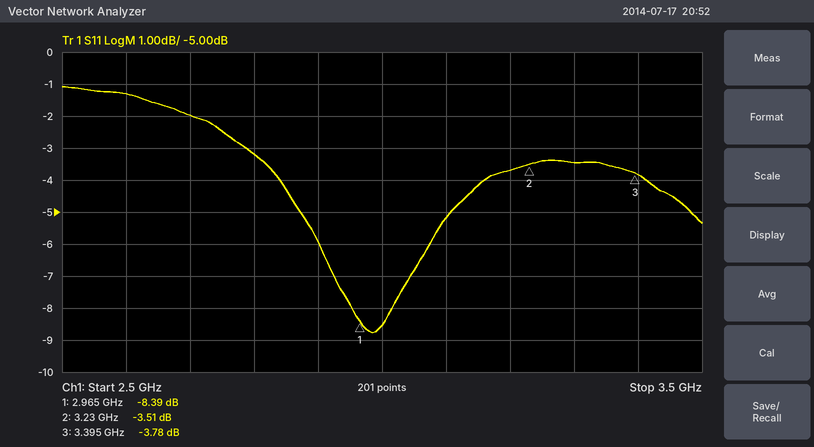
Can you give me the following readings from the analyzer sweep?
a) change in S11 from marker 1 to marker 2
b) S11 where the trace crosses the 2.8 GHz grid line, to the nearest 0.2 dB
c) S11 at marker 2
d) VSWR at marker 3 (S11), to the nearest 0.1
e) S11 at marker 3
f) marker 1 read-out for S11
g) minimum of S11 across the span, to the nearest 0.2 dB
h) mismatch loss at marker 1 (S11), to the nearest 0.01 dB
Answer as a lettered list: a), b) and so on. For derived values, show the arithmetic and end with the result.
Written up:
a) -3.51 − (-8.39) = 4.88 dB
b) -3.2 dB
c) -3.51 dB
d) (1 + 0.6471)/(1 − 0.6471) ≈ 4.7
e) -3.78 dB
f) -8.39 dB
g) -8.8 dB
h) −10 log10(1 − 10^(-8.39/10)) ≈ 0.68 dB
